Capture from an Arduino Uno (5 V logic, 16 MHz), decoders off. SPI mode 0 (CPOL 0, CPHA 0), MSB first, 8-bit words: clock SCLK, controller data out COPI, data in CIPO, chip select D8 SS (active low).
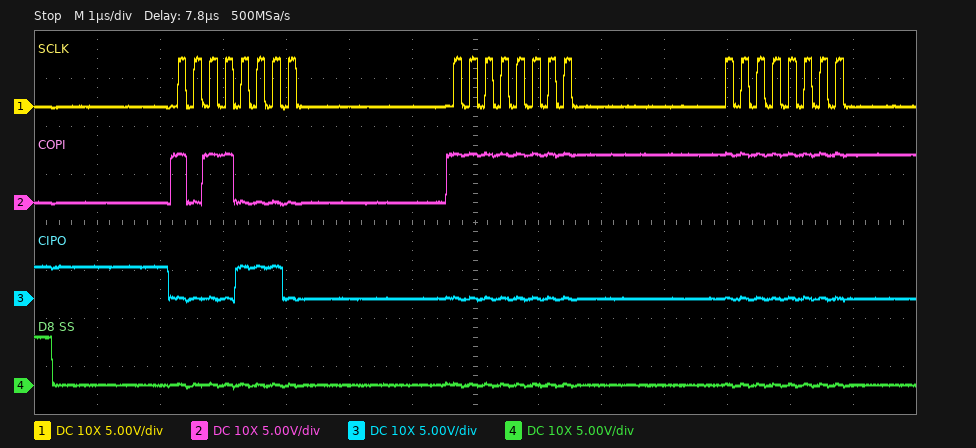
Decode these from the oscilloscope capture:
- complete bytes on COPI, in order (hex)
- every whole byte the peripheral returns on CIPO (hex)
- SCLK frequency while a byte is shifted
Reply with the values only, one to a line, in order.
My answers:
B0 FF FF
0E 00 00
4 MHz
